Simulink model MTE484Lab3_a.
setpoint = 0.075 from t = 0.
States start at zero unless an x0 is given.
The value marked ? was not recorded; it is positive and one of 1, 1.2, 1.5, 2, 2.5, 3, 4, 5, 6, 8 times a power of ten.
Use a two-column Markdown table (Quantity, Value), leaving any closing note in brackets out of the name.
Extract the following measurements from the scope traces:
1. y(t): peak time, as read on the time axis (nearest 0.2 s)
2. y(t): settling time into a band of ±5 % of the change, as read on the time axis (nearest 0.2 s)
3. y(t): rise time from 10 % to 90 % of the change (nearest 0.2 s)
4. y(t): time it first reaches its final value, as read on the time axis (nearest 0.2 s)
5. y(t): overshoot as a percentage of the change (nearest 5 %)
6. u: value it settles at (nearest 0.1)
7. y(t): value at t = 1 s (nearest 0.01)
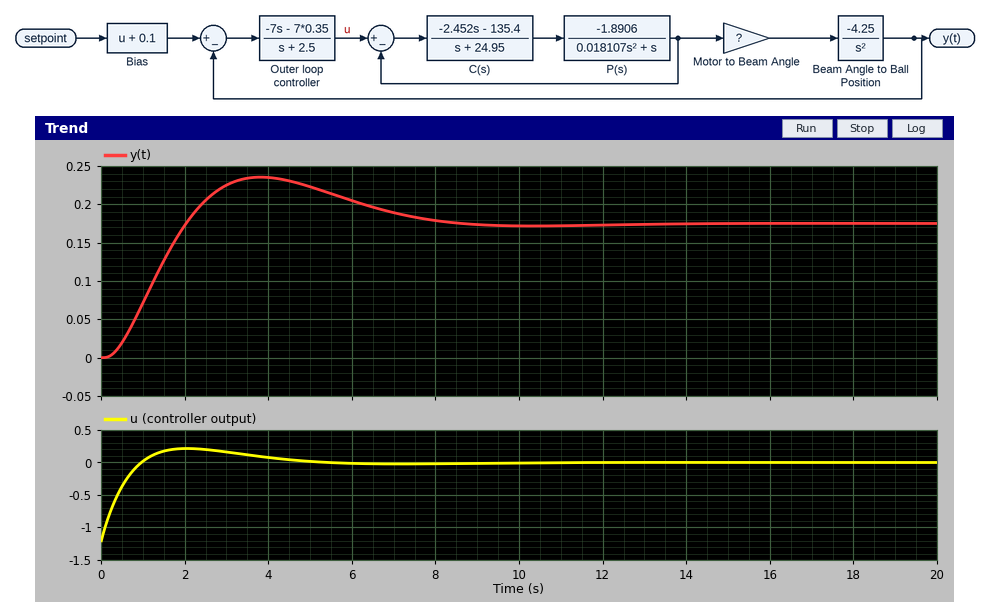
| Quantity | Value |
|---|---|
| y(t): peak time, as read on the time axis | 3.8 s |
| y(t): settling time into a band of ±5 % of the change, as read on the time axis | 7.4 s |
| y(t): rise time from 10 % to 90 % of the change | 1.4 s |
| y(t): time it first reaches its final value, as read on the time axis | 2.0 s |
| y(t): overshoot as a percentage of the change | 35 % |
| u: value it settles at | 0.0 |
| y(t): value at t = 1 s | 0.07 |
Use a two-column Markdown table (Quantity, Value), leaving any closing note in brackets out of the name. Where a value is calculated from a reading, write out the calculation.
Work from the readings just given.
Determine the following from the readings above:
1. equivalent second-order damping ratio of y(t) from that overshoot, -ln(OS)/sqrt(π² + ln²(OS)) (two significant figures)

| Quantity | Value |
|---|---|
| equivalent second-order damping ratio of y(t) from that overshoot, -ln(OS)/sqrt(π² + ln²(OS)) | ln(0.35) = -1.050; 1.050 / sqrt(9.870 + 1.102) = 0.32 |
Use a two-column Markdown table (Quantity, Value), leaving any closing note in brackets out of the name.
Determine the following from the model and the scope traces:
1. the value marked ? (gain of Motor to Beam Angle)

| Quantity | Value |
|---|---|
| the value marked ? | 0.06 |
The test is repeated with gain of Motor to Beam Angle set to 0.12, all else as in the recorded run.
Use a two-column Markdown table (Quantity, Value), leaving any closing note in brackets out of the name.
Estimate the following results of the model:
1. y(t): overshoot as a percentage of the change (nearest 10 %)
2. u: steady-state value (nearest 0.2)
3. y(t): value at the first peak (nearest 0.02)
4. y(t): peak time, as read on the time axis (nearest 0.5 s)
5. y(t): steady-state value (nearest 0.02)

| Quantity | Value |
|---|---|
| y(t): overshoot as a percentage of the change | 40 % |
| u: steady-state value | 0.0 |
| y(t): value at the first peak | 0.24 |
| y(t): peak time, as read on the time axis | 2.0 s |
| y(t): steady-state value | 0.18 |
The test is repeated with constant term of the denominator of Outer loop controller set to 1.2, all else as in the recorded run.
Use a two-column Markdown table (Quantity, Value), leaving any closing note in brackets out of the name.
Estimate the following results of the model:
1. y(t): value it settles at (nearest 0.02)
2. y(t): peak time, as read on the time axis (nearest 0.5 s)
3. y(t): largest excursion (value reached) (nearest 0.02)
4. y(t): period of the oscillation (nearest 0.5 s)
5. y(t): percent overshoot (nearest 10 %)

| Quantity | Value |
|---|---|
| y(t): value it settles at | 0.18 |
| y(t): peak time, as read on the time axis | 2.5 s |
| y(t): largest excursion (value reached) | 0.28 |
| y(t): period of the oscillation | 5.5 s |
| y(t): percent overshoot | 60 % |
